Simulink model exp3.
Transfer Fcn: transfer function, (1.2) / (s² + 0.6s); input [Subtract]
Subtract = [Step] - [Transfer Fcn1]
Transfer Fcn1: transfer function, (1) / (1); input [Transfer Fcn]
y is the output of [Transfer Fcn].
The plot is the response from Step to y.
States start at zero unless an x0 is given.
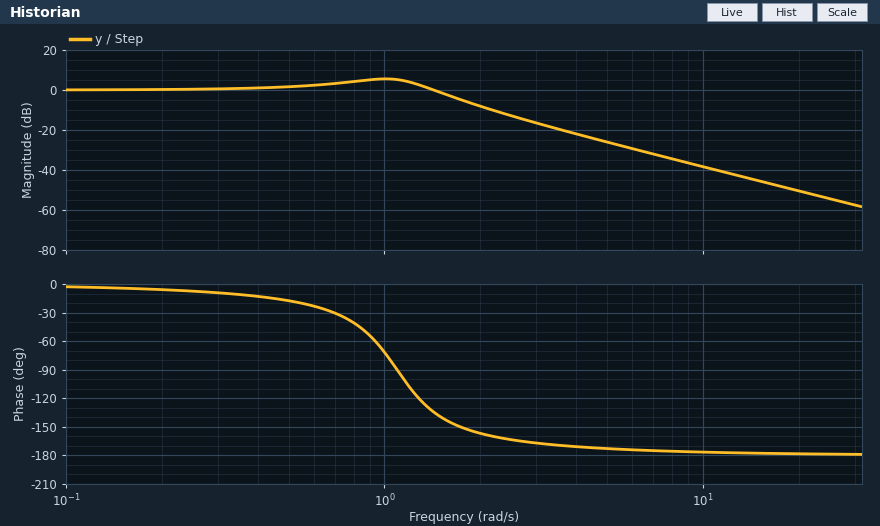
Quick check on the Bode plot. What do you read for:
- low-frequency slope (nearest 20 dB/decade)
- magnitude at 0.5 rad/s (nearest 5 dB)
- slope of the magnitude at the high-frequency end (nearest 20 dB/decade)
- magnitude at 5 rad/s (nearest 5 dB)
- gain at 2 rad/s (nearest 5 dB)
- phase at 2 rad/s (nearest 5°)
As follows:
0 dB/decade
0 dB
-40 dB/decade
-25 dB
-10 dB
-155°
